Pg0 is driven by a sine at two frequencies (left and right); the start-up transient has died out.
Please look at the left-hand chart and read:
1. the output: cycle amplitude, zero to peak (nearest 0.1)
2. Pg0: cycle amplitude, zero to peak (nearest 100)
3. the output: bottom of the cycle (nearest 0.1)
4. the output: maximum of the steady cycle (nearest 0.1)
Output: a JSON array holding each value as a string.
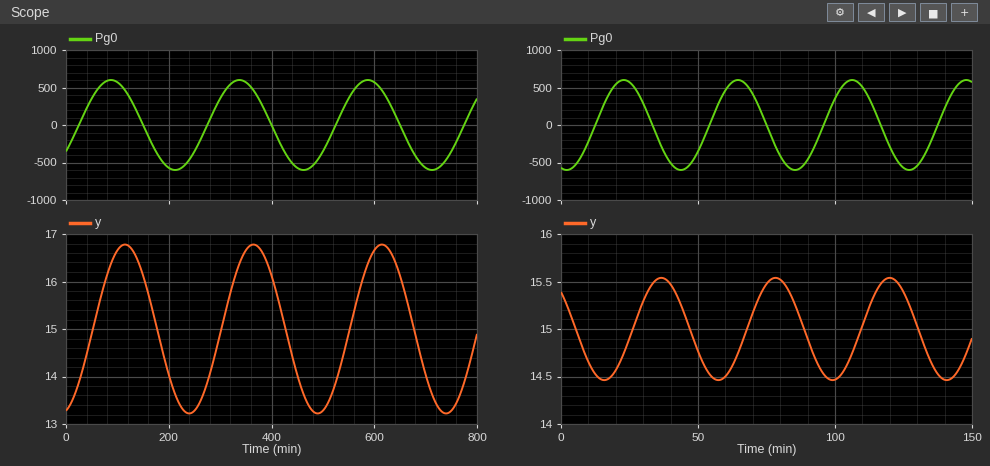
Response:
["1.8", "600", "13.2", "16.8"]
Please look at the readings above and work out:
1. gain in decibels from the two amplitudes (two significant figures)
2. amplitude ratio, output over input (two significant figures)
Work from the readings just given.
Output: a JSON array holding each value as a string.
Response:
["-50 dB", "0.0030"]
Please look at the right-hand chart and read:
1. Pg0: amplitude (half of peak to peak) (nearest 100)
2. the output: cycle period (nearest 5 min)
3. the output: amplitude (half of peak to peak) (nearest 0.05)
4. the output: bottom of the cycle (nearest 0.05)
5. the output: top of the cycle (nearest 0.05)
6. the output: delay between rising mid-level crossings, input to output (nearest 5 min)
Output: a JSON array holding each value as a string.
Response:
["600", "40 min", "0.55", "14.45", "15.55", "15 min"]
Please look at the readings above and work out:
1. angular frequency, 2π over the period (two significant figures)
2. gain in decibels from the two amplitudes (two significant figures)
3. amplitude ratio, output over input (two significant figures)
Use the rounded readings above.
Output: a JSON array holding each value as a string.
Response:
["0.16 rad/min", "-61 dB", "0.00092"]
